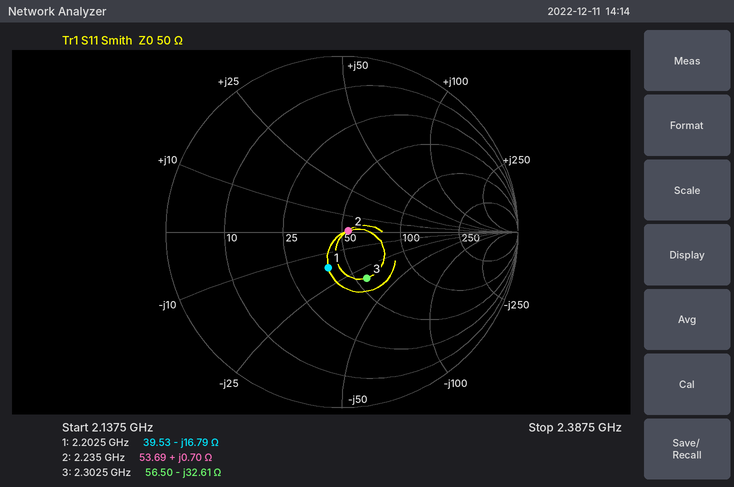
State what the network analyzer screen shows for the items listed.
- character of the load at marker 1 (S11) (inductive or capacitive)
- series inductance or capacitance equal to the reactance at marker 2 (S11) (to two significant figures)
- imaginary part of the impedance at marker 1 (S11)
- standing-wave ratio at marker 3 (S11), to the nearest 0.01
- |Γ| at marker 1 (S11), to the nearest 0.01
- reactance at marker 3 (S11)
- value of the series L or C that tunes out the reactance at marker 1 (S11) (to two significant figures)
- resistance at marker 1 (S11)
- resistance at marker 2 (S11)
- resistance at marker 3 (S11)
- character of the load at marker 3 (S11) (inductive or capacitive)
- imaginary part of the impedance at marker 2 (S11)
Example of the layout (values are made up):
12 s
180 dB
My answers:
capacitive
50 pH
-16.79 Ω
1.85
0.22
-32.61 Ω
1.2 nH
39.53 Ω
53.69 Ω
56.50 Ω
capacitive
+0.70 Ω
